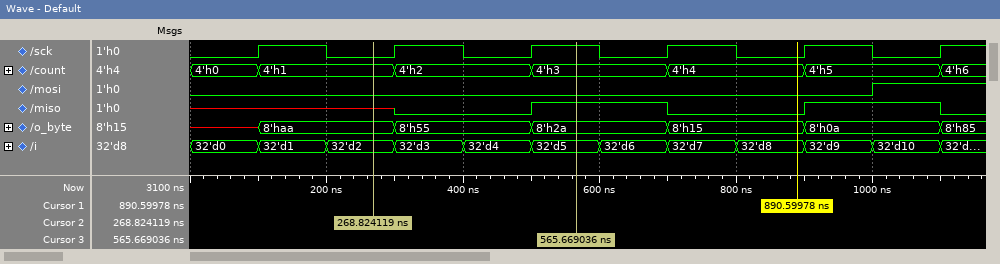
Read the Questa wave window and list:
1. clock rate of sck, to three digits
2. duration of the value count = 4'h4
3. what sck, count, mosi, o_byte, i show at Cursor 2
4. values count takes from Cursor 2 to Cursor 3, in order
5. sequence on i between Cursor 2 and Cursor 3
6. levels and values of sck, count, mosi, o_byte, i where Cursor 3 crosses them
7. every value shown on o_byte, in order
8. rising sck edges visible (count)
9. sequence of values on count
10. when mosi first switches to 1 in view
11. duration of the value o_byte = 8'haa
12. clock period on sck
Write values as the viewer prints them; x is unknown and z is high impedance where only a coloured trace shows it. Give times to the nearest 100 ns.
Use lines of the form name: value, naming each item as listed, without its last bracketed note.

clock rate of sck, to three digits: 5.00 MHz
duration of the value count = 4'h4: 200 ns
what sck, count, mosi, o_byte, i show at Cursor 2: sck=0, count=4'h1, mosi=0, o_byte=8'haa, i=32'd2
values count takes from Cursor 2 to Cursor 3, in order: 4'h1, 4'h2, 4'h3
sequence on i between Cursor 2 and Cursor 3: 32'd2, 32'd3, 32'd4, 32'd5
levels and values of sck, count, mosi, o_byte, i where Cursor 3 crosses them: sck=1, count=4'h3, mosi=0, o_byte=8'h2a, i=32'd5
every value shown on o_byte, in order: x, 8'haa, 8'h55, 8'h2a, 8'h15, 8'h0a, 8'h85
rising sck edges visible: 6
sequence of values on count: 4'h0, 4'h1, 4'h2, 4'h3, 4'h4, 4'h5, 4'h6
when mosi first switches to 1 in view: 1000 ns
duration of the value o_byte = 8'haa: 200 ns
clock period on sck: 200 ns
